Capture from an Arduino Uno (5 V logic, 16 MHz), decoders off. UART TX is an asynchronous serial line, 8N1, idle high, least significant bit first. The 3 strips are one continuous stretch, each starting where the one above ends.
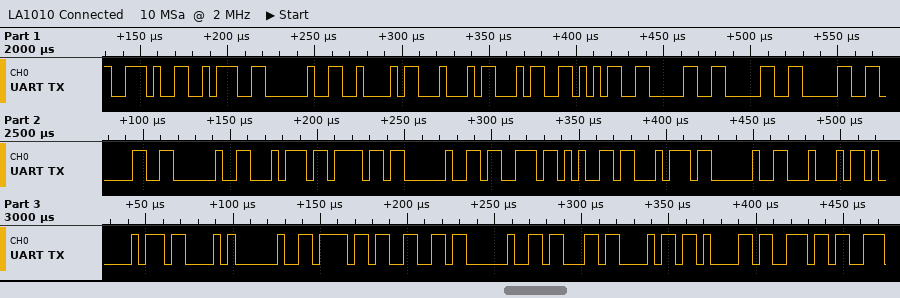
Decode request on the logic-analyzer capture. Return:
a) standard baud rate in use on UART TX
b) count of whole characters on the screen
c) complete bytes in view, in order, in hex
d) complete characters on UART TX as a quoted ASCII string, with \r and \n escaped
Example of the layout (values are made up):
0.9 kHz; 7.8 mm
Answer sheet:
250000 baud; 30; 2E 3A 20 42 44 34 35 30 30 30 30 20 74 6F 20 73 65 74 20 44 41 43 20 6F 66 20 63 68 61 6E; ".: BD450000 to set DAC of chan"
